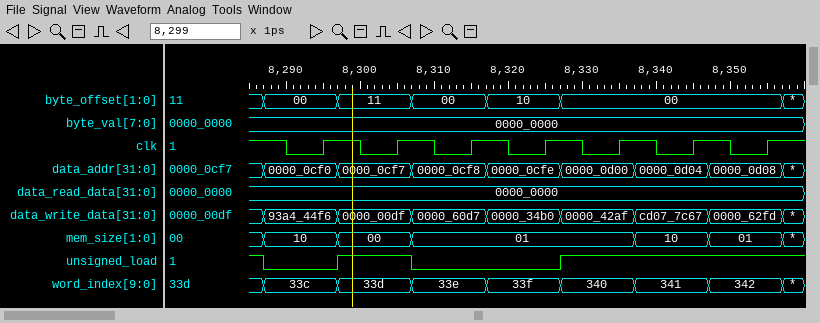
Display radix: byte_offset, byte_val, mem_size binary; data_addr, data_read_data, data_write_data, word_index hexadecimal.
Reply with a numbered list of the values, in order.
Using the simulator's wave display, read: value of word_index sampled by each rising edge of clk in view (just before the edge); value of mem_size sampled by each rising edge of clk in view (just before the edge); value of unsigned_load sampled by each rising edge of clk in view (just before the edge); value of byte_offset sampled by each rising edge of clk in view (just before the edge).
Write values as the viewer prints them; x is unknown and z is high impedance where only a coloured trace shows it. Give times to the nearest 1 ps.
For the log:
1. 33c, 33d, 33e, 33f, 340, 341, 342
2. 10, 00, 01, 01, 01, 10, 01
3. 0 1 0 0 1 1 1
4. 00, 11, 00, 10, 00, 00, 00
